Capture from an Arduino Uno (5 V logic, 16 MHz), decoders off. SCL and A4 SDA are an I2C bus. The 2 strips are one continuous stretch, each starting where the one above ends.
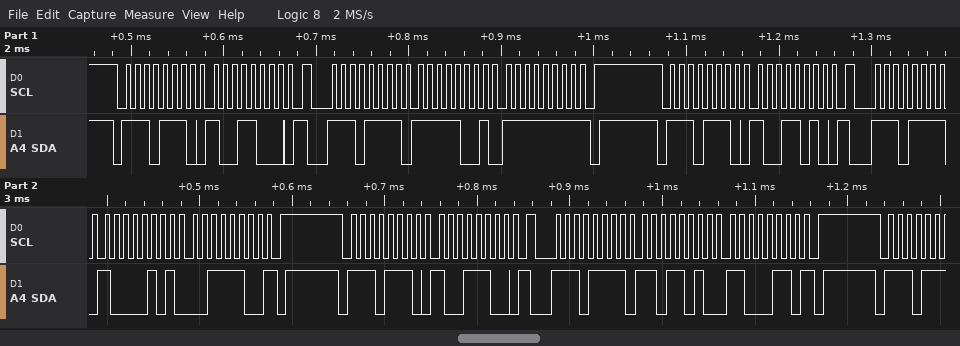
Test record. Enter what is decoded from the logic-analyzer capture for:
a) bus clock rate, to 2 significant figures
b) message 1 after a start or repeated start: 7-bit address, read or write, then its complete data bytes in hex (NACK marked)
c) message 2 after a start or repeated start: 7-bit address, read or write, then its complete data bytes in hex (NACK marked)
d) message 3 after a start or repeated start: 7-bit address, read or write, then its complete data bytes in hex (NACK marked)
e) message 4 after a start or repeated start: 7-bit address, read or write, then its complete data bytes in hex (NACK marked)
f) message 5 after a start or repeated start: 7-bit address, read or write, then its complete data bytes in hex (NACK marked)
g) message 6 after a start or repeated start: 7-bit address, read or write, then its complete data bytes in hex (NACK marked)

100 kHz
0x77 write: 98
0x77 read: F9 FF NACK
0x77 write: 9A
0x77 read: 85 3C NACK
0x77 write: 9C
0x77 read: DA C6 NACK
